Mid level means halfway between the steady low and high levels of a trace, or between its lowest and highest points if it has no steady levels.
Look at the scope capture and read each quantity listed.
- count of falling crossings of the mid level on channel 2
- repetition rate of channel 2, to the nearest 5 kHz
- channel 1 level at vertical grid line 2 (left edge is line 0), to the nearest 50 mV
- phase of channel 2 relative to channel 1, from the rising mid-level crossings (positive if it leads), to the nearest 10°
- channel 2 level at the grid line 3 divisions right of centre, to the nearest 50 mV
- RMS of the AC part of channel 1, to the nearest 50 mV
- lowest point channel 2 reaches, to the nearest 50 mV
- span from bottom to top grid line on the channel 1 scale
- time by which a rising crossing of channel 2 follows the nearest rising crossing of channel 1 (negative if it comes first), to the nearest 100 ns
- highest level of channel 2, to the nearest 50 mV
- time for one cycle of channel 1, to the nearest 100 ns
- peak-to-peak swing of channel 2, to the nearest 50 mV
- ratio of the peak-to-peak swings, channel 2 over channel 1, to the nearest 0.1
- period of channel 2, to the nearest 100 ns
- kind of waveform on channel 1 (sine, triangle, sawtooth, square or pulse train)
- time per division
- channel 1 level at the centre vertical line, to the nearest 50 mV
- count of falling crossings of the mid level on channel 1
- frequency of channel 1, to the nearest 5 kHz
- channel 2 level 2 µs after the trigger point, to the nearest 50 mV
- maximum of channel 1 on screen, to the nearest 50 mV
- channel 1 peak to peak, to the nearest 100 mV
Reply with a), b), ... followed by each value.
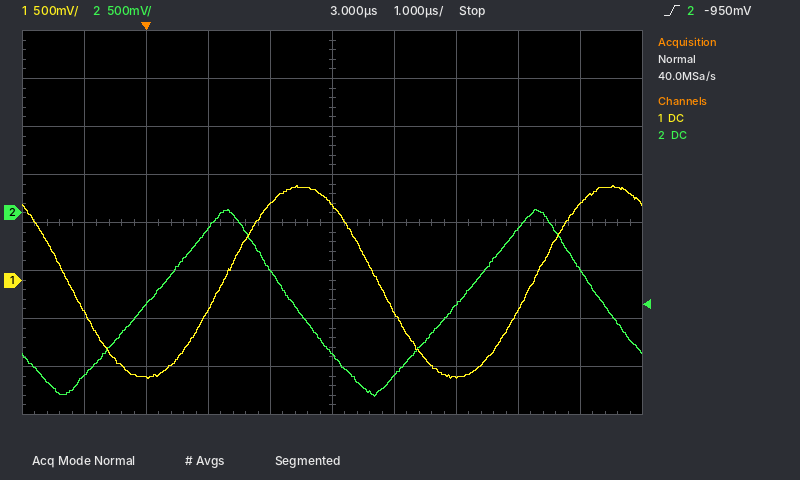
a) 2
b) 200 kHz
c) -1.00 V
d) +90°
e) -150 mV
f) 700 mV
g) -1.90 V
h) 4 V
i) -1.2 µs
j) 50 mV
k) 5.0 µs
l) 1.95 V
m) 1.0
n) 5.0 µs
o) sine
p) 1 µs
q) 800 mV
r) 2
s) 200 kHz
t) -600 mV
u) 1.00 V
v) 2.00 V
